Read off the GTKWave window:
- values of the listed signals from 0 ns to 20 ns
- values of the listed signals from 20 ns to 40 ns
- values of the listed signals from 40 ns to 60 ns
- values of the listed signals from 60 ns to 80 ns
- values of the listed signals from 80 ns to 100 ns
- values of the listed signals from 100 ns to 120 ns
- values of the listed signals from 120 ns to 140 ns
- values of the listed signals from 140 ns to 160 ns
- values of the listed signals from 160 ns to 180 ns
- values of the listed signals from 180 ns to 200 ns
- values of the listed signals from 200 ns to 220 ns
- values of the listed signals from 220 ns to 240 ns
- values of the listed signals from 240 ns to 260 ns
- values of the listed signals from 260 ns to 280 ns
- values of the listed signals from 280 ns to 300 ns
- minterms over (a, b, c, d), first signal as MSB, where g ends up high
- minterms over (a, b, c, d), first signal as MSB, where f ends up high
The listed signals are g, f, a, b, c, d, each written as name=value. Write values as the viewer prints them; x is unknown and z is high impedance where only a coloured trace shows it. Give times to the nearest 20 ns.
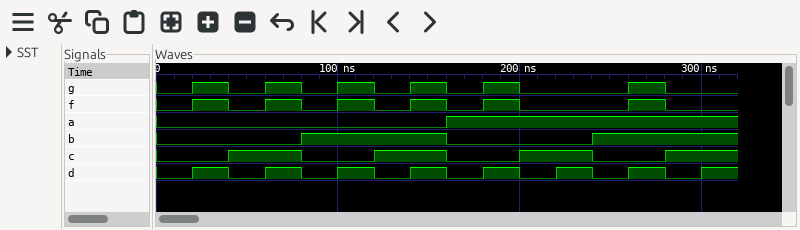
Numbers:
g=0, f=0, a=0, b=0, c=0, d=0
g=1, f=1, a=0, b=0, c=0, d=1
g=0, f=0, a=0, b=0, c=1, d=0
g=1, f=1, a=0, b=0, c=1, d=1
g=0, f=0, a=0, b=1, c=0, d=0
g=1, f=1, a=0, b=1, c=0, d=1
g=0, f=0, a=0, b=1, c=1, d=0
g=1, f=1, a=0, b=1, c=1, d=1
g=0, f=0, a=1, b=0, c=0, d=0
g=1, f=1, a=1, b=0, c=0, d=1
g=0, f=0, a=1, b=0, c=1, d=0
g=0, f=0, a=1, b=0, c=1, d=1
g=0, f=0, a=1, b=1, c=0, d=0
g=1, f=1, a=1, b=1, c=0, d=1
g=0, f=0, a=1, b=1, c=1, d=0
1, 3, 5, 7, 9, 13
1, 3, 5, 7, 9, 13
